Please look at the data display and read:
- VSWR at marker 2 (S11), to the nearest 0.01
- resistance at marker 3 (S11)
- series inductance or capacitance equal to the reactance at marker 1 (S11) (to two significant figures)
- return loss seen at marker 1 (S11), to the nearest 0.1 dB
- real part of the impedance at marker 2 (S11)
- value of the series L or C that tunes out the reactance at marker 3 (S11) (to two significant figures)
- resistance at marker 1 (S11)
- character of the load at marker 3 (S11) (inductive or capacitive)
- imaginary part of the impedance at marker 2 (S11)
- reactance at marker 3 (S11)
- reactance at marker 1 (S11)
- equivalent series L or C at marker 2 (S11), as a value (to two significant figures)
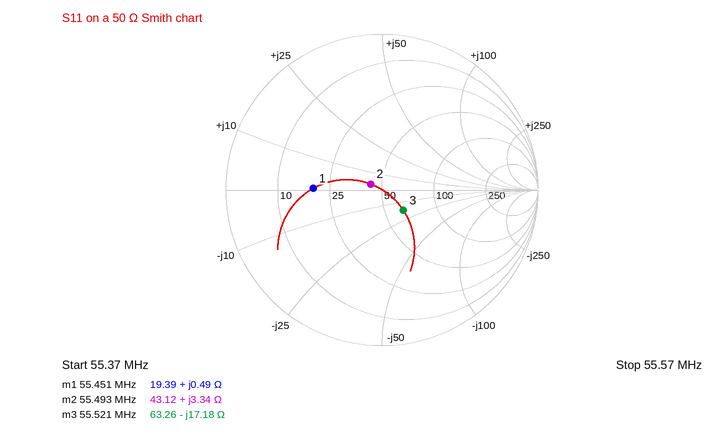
1.18
63.26 Ω
1.4 nH
7.1 dB
43.12 Ω
49 nH
19.39 Ω
capacitive
+3.34 Ω
-17.18 Ω
+0.49 Ω
9.6 nH
